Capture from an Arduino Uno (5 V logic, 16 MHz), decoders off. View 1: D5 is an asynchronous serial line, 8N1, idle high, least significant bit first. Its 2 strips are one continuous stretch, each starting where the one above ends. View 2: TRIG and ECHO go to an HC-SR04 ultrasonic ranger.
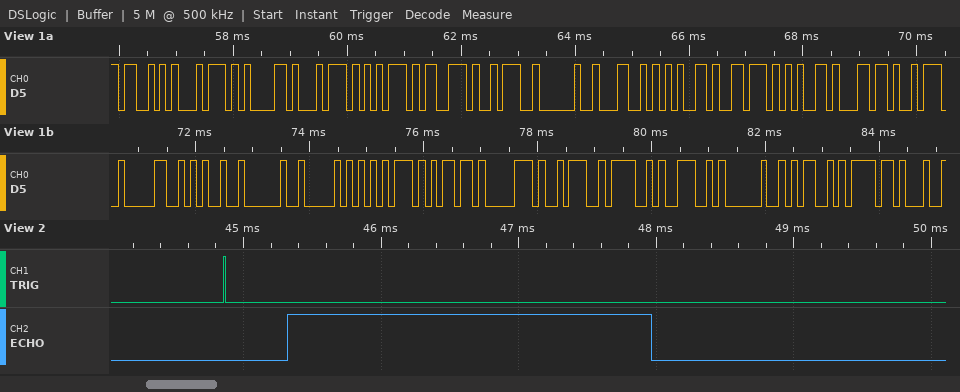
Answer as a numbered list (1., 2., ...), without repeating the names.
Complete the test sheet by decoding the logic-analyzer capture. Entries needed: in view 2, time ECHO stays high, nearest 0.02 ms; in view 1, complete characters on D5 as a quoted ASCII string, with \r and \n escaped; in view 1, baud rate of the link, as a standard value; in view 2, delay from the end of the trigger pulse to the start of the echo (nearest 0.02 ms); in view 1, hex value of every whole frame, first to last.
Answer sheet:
1. 2.64 ms
2. "Status: Level:0% Pump:ON Mo"
3. 9600 baud
4. 0.46 ms
5. 53 74 61 74 75 73 3A 20 4C 65 76 65 6C 3A 30 25 20 50 75 6D 70 3A 4F 4E 20 4D 6F
